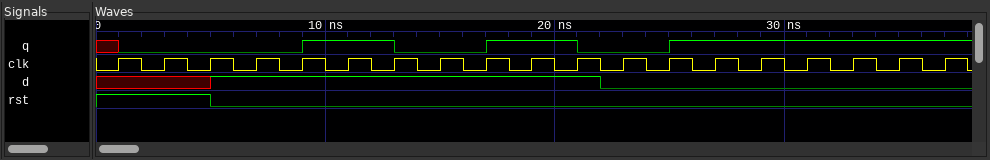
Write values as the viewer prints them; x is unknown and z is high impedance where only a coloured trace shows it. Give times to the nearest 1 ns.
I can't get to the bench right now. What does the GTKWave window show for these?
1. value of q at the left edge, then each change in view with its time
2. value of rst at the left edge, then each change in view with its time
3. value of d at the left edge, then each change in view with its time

x, 0 at 1 ns, 1 at 9 ns, 0 at 13 ns, 1 at 17 ns, 0 at 21 ns, 1 at 25 ns
1, 0 at 5 ns
x, 1 at 5 ns, 0 at 22 ns
